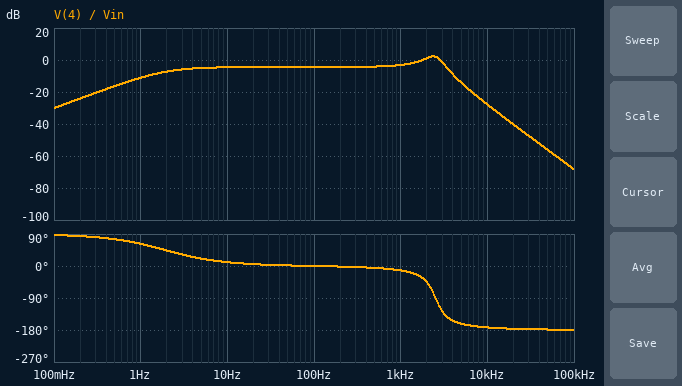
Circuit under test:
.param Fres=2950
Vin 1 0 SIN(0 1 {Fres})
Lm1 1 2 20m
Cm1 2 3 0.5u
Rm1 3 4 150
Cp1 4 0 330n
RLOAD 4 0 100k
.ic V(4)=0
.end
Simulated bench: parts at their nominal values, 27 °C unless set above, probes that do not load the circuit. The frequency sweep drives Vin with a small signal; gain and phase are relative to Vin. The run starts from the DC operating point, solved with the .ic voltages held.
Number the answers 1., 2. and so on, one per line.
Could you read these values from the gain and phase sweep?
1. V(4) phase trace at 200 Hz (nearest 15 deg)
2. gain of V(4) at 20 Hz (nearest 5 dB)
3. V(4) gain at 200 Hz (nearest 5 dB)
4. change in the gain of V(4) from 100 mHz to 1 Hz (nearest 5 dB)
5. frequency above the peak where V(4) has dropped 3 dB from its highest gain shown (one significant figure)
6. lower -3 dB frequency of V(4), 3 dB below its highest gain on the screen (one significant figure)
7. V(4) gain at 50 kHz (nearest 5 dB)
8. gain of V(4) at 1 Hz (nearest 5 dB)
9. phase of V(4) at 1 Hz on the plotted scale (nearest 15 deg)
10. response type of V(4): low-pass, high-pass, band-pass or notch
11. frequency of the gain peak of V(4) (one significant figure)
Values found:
1. 0 deg
2. -5 dB
3. -5 dB
4. 20 dB
5. 3 kHz
6. 2 kHz
7. -55 dB
8. -10 dB
9. 60 deg
10. band-pass
11. 2 kHz
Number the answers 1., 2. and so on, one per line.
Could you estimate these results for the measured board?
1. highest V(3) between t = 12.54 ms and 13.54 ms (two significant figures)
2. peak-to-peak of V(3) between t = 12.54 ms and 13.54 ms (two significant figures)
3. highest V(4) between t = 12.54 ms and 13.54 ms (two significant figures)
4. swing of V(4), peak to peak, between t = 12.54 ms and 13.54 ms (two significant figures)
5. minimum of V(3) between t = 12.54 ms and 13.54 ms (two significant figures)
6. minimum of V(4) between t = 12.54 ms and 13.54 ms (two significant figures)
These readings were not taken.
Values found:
1. 1.2 V
2. 2.5 V
3. 910 mV
4. 1.8 V
5. -1.2 V
6. -910 mV
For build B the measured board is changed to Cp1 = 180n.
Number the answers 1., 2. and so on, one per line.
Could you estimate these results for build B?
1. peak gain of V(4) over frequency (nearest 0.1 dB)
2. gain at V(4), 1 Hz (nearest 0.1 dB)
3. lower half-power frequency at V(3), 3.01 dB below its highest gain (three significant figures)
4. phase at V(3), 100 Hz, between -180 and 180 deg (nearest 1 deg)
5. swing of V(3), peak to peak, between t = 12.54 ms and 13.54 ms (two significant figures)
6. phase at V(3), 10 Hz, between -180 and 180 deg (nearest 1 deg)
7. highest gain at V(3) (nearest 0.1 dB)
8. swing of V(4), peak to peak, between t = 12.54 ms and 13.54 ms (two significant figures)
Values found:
1. 5.7 dB
2. -10.8 dB
3. 2.35 kHz
4. 2 deg
5. 4.3 V
6. 13 deg
7. 6.7 dB
8. 3.9 V
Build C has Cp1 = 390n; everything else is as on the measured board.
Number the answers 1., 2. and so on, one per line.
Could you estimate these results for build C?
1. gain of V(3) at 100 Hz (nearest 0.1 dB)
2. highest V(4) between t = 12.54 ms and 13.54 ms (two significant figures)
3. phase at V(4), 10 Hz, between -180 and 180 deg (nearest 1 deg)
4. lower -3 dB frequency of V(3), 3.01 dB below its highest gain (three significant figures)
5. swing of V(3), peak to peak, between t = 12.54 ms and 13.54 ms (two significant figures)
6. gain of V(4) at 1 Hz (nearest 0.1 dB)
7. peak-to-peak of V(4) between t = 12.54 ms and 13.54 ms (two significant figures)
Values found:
1. -5.0 dB
2. 710 mV
3. 10 deg
4. 1.69 kHz
5. 2.1 V
6. -11.2 dB
7. 1.4 V
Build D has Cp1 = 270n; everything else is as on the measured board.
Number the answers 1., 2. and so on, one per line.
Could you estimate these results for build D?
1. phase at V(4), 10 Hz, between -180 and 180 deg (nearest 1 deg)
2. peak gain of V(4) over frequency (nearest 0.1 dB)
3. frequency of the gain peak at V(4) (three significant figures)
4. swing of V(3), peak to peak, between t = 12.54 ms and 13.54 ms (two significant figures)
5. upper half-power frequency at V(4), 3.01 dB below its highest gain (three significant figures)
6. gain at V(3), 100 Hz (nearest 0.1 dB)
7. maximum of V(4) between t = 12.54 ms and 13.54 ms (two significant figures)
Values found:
1. 12 deg
2. 3.5 dB
3. 2.55 kHz
4. 3.1 V
5. 3.11 kHz
6. -3.7 dB
7. 1.2 V
